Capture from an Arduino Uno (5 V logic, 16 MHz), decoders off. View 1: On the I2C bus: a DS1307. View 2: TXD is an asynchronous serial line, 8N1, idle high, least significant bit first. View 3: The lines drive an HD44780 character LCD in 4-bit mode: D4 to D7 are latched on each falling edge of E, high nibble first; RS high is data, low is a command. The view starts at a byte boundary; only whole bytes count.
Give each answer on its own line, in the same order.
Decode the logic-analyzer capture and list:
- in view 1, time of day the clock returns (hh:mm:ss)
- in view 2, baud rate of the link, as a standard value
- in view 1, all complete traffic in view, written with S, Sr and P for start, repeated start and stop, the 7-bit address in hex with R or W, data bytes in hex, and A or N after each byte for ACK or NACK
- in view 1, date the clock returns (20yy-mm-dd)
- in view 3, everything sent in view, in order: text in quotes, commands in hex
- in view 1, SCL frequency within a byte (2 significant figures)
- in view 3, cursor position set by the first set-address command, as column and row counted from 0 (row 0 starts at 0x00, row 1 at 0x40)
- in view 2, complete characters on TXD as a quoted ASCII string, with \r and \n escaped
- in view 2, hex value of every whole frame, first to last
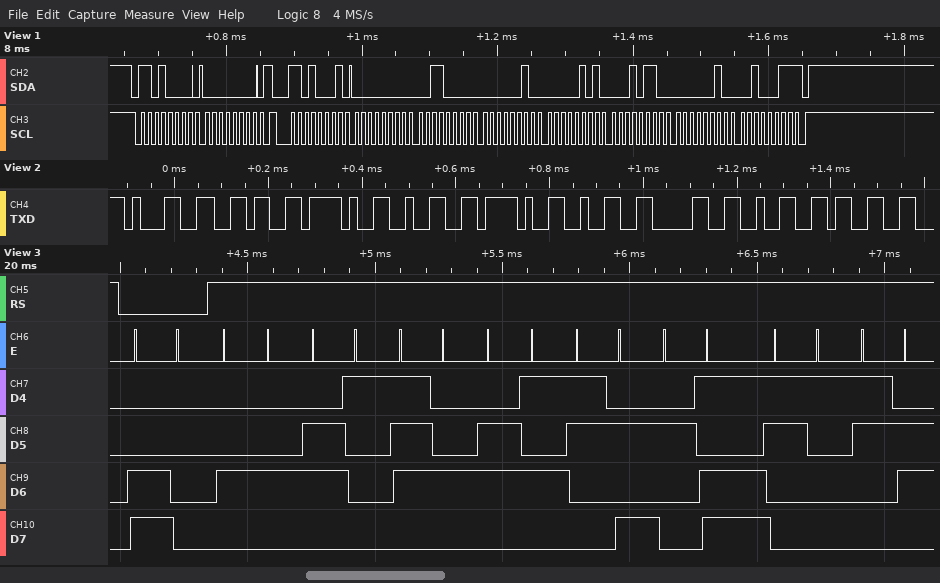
02:30:00
57600 baud
S 68W A 00 A Sr 68R A 00 A 30 A 02 A 05 A 16 A 02 A 23 N P
2023-02-16
0xC0 "Date:-16"
100 kHz
column 0, row 1
"16/2/2023"
31 36 2F 32 2F 32 30 32 33
